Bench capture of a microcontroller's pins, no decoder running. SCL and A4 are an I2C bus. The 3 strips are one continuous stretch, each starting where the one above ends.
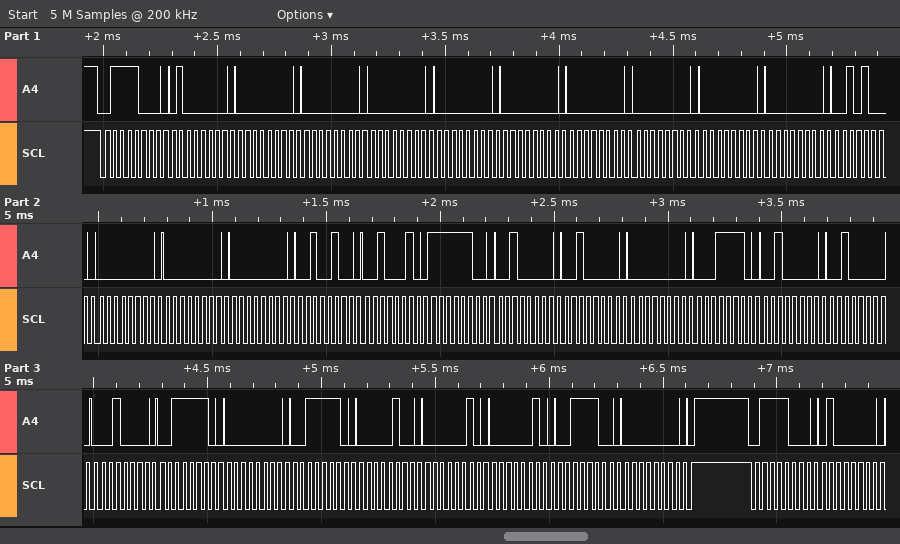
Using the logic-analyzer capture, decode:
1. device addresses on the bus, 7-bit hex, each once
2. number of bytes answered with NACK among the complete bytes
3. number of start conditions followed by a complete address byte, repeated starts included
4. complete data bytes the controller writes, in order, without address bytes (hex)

0x3C
0
2
40 00 00 00 00 00 00 00 00 00 28 00 00 00 24 22 FC 20 20 00 1E 20 20 10 3E 00 3E 04 02 02 3C 00 40
